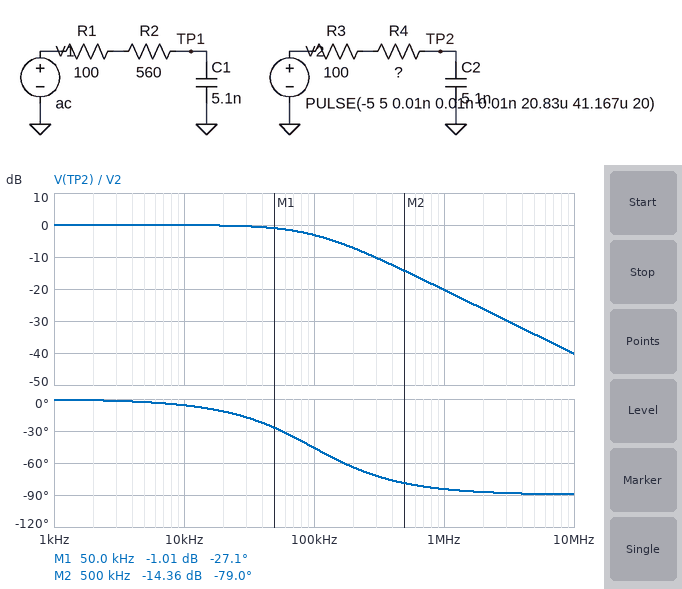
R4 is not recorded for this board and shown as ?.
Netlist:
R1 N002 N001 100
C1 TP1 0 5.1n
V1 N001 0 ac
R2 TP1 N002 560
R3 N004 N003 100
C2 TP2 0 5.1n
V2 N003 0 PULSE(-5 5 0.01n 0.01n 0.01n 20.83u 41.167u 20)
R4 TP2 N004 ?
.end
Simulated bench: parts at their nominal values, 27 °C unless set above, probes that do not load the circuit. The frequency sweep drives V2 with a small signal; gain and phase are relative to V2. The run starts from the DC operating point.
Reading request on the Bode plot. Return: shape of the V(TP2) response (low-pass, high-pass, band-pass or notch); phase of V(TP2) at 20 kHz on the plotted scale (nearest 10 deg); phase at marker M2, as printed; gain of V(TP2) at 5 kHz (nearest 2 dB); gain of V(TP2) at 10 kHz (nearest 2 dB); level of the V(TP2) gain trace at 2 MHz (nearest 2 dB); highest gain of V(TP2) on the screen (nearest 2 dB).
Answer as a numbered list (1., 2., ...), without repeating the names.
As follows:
1. low-pass
2. -10 deg
3. -79.0 deg
4. 0 dB
5. 0 dB
6. -26 dB
7. 0 dB
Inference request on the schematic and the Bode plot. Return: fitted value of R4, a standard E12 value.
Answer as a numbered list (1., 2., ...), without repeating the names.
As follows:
1. 220 Ω
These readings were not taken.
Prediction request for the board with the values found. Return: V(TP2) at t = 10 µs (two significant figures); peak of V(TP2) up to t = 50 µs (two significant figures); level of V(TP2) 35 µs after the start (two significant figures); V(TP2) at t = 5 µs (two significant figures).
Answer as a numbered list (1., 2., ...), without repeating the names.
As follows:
1. 5.0 V
2. 5.0 V
3. -5.0 V
4. 4.5 V
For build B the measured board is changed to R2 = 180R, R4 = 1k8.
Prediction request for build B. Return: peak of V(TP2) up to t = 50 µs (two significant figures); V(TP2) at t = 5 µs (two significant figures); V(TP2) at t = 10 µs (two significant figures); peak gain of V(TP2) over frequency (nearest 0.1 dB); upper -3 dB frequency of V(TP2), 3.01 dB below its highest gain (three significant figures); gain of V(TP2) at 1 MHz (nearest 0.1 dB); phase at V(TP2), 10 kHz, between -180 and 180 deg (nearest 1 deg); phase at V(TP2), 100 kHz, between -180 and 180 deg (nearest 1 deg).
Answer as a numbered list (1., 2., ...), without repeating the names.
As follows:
1. 3.8 V
2. -970 mV
3. 1.4 V
4. 0 dB
5. 16.4 kHz
6. -35.7 dB
7. -31 deg
8. -81 deg
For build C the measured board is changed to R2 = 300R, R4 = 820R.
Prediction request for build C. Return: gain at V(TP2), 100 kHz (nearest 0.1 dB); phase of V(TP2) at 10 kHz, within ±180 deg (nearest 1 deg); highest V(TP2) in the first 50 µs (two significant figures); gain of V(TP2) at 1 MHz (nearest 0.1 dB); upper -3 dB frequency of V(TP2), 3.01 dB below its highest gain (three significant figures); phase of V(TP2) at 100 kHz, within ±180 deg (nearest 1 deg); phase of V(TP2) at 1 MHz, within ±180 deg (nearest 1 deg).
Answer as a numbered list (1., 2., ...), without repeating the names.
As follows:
1. -9.9 dB
2. -16 deg
3. 4.9 V
4. -29.4 dB
5. 33.9 kHz
6. -71 deg
7. -88 deg
